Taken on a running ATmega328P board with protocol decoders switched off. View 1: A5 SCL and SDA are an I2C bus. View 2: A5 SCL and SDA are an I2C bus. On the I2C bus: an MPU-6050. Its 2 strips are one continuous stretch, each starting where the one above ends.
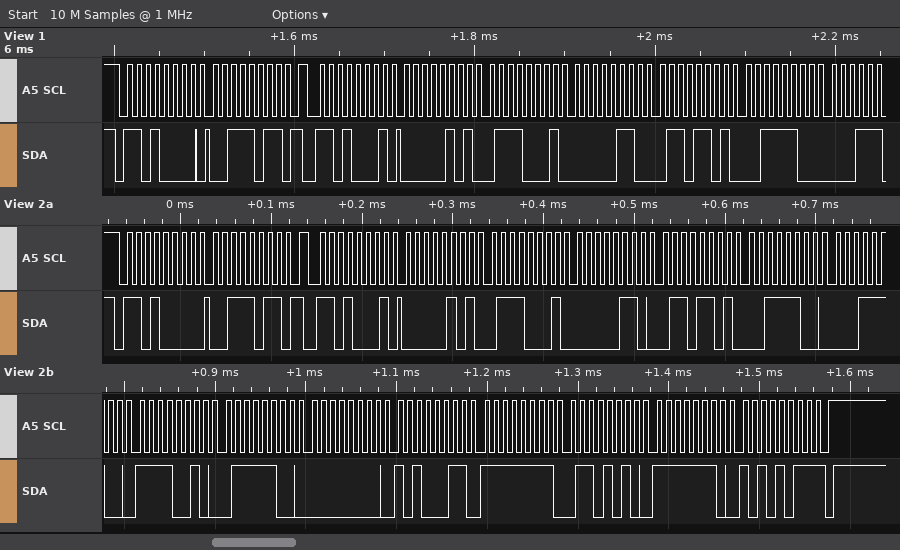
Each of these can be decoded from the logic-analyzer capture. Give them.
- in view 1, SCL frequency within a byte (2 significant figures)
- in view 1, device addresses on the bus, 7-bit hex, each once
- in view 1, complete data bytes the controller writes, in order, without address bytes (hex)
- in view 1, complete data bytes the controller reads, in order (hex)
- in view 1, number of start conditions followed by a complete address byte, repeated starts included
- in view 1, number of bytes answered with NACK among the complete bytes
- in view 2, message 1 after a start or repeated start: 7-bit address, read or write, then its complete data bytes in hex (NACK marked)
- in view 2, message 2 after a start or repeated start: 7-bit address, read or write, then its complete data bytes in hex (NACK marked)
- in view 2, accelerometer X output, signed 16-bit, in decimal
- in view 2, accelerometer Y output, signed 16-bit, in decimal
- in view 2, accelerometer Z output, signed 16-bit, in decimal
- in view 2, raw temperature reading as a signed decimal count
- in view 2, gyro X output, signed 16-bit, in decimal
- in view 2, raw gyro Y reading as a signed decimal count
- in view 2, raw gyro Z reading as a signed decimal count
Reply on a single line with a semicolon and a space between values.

100 kHz; 0x68; 3B; 05 71 06 6D 3C; 2; 0; 0x68 write: 3B; 0x68 read: 05 71 06 6D 3C 1C F2 7C 00 A3 FF 6A FE AB NACK; 1393; 1645; 15388; -3460; 163; -150; -341
